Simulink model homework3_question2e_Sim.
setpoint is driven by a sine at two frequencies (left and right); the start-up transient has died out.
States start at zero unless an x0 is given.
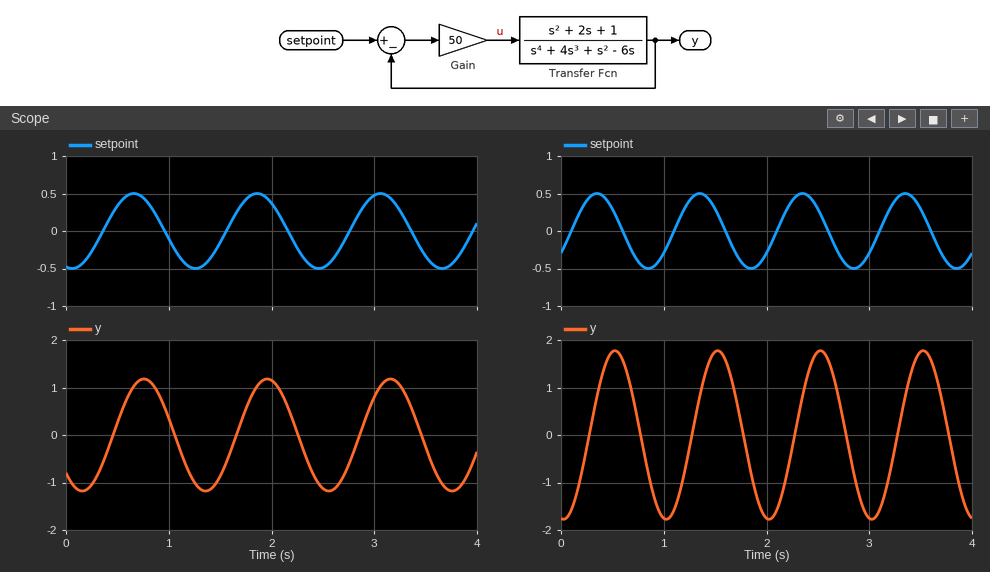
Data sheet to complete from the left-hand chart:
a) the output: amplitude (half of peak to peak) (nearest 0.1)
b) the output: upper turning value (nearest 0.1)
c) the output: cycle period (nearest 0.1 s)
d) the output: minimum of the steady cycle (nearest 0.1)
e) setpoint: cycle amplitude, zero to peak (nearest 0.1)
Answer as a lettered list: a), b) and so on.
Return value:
a) 1.2
b) 1.2
c) 1.2 s
d) -1.2
e) 0.5
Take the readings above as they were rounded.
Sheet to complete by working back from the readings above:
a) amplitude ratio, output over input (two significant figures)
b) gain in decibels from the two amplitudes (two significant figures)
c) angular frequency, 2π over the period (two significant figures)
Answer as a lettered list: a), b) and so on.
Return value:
a) 2.4
b) 7.6 dB
c) 5.2 rad/s
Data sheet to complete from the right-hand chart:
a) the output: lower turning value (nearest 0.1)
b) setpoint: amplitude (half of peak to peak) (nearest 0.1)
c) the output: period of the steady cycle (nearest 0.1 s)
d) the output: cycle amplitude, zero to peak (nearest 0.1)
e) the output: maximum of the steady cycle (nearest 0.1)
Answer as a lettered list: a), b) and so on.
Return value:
a) -1.8
b) 0.5
c) 1.0 s
d) 1.8
e) 1.8
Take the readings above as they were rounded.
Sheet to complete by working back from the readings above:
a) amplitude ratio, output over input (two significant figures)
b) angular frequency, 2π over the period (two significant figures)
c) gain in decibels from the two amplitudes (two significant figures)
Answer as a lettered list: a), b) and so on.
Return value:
a) 3.6
b) 6.3 rad/s
c) 11 dB
